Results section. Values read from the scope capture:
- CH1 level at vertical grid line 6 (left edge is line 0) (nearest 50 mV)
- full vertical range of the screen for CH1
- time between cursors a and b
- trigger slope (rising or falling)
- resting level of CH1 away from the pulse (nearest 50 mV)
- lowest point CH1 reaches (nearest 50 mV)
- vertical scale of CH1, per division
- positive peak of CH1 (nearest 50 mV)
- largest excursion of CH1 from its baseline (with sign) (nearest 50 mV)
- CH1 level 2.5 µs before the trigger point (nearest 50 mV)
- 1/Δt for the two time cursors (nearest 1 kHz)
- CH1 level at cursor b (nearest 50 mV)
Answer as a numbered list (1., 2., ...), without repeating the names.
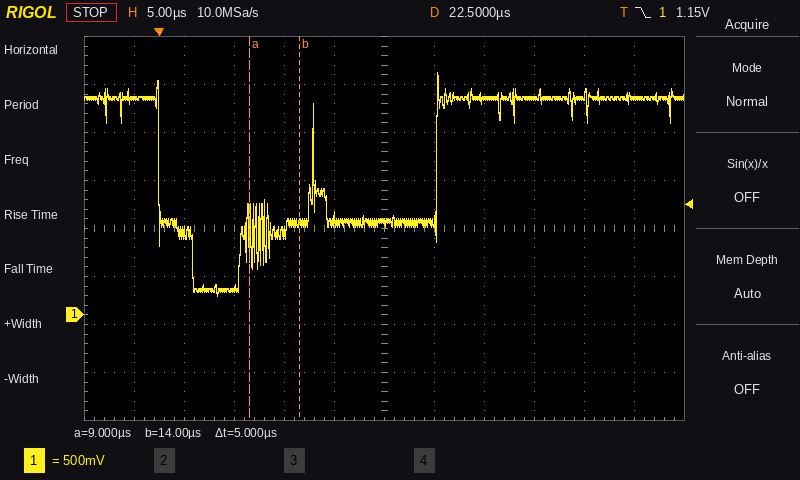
1. 950 mV
2. 4 V
3. 5 µs
4. falling
5. 2.25 V
6. 200 mV
7. 500 mV
8. 2.50 V
9. -2.05 V
10. 2.25 V
11. 200 kHz
12. 950 mV
